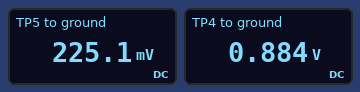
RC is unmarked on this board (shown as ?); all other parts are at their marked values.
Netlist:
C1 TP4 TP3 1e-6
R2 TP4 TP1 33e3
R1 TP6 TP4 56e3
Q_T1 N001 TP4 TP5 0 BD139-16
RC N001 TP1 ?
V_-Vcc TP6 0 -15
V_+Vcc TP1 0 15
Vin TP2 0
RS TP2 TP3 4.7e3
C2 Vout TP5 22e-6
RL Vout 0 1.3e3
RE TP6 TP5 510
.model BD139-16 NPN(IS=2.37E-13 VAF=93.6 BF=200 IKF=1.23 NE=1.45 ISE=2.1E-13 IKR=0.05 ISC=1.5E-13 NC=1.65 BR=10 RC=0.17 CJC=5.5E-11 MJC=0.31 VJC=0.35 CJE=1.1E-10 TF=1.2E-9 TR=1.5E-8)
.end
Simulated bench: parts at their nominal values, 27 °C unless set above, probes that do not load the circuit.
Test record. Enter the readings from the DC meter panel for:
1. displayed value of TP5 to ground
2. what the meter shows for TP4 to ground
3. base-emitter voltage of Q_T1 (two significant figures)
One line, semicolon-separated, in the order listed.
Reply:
225.1 mV; 0.884 V; 660 mV
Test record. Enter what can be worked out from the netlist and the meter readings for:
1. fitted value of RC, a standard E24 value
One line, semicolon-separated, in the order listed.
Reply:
91 Ω
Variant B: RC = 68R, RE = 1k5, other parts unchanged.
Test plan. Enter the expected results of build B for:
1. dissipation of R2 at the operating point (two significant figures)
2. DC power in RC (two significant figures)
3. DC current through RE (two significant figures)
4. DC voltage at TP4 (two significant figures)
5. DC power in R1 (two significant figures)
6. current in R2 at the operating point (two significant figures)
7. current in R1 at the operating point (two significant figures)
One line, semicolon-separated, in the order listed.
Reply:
4.6 mW; 8.7 mW; 11 mA; 2.7 V; 5.6 mW; 370 µA; 320 µA
